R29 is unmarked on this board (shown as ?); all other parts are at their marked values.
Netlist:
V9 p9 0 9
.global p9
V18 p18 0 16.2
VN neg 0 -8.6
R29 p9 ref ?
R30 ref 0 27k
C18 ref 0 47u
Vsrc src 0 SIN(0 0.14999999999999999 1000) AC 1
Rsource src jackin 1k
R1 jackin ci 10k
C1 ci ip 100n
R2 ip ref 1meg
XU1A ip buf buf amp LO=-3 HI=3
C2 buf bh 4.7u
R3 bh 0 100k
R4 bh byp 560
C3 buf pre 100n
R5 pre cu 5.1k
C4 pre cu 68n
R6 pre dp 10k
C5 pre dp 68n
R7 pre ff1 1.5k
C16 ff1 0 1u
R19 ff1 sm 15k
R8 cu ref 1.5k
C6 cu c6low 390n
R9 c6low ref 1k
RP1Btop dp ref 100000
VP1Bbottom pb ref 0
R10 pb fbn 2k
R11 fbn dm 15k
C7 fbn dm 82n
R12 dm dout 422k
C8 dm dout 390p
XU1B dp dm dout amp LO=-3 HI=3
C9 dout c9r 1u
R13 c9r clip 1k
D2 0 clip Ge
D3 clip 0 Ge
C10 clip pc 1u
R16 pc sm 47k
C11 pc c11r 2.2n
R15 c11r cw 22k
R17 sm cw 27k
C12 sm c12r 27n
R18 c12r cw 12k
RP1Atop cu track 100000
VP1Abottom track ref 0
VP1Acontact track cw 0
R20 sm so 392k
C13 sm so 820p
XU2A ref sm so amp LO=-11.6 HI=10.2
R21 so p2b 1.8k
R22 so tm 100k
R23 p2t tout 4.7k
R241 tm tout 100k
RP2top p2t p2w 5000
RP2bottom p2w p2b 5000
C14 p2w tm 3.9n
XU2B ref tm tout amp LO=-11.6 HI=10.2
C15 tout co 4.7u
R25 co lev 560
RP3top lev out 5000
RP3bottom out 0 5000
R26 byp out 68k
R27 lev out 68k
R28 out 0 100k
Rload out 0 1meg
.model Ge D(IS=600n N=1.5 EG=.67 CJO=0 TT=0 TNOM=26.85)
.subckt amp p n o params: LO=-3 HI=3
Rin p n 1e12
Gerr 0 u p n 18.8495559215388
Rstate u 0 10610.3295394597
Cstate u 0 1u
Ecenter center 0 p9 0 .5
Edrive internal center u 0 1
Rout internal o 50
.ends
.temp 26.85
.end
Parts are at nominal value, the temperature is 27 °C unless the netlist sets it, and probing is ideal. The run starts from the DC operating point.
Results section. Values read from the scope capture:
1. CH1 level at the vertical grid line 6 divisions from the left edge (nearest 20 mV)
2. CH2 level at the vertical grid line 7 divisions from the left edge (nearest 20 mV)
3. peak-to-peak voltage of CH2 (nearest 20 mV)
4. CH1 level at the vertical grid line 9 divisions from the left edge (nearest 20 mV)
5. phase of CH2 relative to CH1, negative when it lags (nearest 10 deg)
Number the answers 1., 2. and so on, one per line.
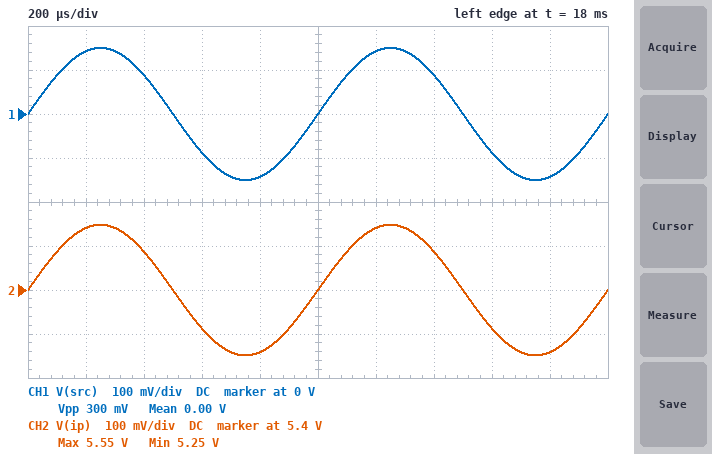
1. 140 mV
2. 5.48 V
3. 300 mV
4. -140 mV
5. 0 deg
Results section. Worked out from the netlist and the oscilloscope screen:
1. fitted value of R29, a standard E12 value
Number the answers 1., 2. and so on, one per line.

1. 18 kΩ
